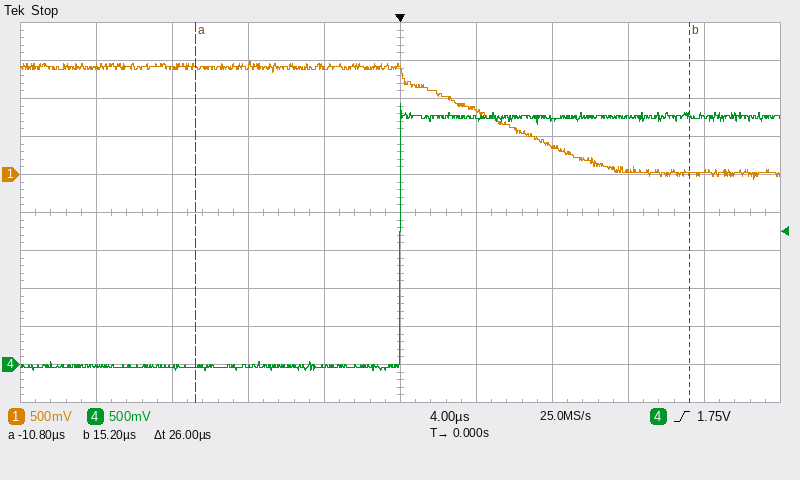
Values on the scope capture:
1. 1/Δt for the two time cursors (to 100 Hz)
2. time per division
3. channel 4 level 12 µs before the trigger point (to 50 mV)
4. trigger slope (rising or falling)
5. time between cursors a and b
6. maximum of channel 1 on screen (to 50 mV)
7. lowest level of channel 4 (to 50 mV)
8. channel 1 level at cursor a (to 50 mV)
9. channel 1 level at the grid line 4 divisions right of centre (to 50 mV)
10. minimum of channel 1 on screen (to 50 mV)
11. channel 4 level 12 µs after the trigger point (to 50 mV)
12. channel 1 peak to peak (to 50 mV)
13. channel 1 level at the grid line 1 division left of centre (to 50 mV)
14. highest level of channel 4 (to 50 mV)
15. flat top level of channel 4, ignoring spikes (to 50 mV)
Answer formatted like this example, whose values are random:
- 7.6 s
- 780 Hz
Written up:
- 38.5 kHz
- 4 µs
- -50 mV
- rising
- 26 µs
- 1.50 V
- -100 mV
- 1.40 V
- 50 mV
- -50 mV
- 3.25 V
- 1.55 V
- 1.40 V
- 3.45 V
- 3.25 V
